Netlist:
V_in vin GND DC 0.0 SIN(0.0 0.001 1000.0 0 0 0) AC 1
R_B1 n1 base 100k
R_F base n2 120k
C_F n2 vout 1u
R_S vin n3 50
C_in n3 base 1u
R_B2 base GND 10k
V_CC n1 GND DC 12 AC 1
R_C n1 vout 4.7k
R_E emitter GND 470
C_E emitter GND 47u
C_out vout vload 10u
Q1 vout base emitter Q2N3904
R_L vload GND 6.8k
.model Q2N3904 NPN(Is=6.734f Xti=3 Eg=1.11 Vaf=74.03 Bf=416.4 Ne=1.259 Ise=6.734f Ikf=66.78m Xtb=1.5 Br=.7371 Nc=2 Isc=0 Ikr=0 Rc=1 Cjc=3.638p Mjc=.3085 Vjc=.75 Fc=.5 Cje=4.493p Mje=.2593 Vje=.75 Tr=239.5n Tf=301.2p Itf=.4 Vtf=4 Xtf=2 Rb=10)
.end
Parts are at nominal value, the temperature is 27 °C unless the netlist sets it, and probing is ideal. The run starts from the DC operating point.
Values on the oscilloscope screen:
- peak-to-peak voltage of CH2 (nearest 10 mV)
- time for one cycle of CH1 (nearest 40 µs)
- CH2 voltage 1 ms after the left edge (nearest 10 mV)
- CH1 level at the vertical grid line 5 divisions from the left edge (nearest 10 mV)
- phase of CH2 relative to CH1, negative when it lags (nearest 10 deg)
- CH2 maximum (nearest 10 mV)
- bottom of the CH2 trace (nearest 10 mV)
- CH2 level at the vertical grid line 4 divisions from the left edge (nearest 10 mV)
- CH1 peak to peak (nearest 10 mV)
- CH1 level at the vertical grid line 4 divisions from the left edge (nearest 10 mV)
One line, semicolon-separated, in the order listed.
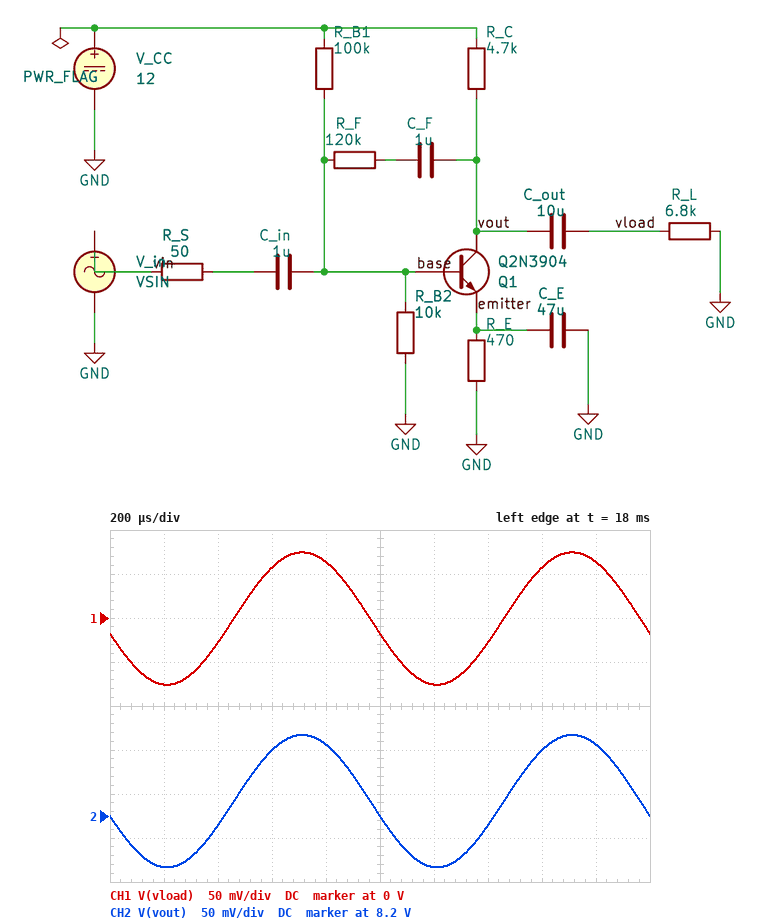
150 mV; 1.00 ms; 8.20 V; -20 mV; 0 deg; 8.29 V; 8.14 V; 8.28 V; 150 mV; 60 mV
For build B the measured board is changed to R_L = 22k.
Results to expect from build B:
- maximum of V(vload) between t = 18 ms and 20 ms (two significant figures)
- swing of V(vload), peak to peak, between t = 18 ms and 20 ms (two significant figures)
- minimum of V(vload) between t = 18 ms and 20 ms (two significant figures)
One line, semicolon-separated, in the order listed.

100 mV; 200 mV; -100 mV
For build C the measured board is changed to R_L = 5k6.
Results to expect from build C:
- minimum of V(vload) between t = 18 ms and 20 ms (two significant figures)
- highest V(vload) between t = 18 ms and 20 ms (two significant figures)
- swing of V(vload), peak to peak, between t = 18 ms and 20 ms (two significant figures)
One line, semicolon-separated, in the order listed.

-70 mV; 69 mV; 140 mV
